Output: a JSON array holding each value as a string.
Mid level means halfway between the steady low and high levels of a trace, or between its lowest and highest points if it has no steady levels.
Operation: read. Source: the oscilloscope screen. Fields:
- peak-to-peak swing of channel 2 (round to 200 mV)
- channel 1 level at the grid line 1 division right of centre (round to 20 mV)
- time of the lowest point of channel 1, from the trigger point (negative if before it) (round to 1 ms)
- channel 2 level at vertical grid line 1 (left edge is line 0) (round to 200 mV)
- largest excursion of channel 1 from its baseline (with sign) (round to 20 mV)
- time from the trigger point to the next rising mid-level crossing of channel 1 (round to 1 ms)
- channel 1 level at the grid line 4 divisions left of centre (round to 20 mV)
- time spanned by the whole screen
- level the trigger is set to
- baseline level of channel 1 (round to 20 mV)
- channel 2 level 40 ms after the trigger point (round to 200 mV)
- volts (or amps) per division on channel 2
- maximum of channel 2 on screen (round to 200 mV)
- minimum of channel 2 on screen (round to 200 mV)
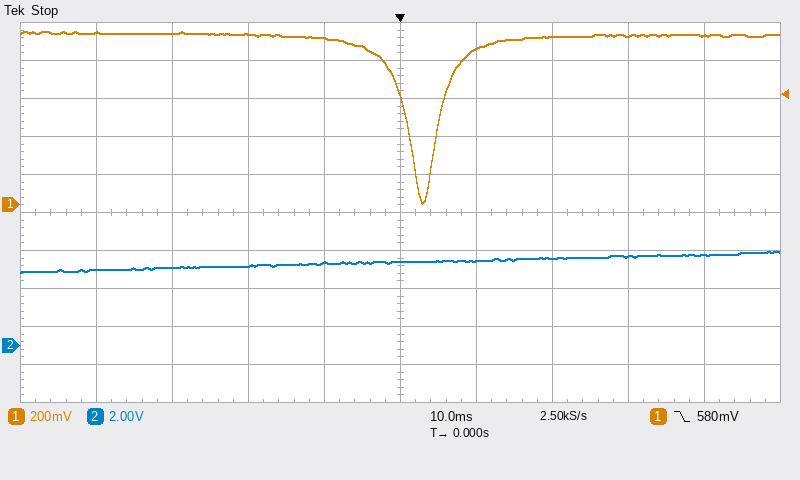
["1.2 V", "820 mV", "+3 ms", "4.0 V", "-880 mV", "5 ms", "900 mV", "100 ms", "580 mV", "900 mV", "4.8 V", "2 V", "5.0 V", "3.8 V"]
